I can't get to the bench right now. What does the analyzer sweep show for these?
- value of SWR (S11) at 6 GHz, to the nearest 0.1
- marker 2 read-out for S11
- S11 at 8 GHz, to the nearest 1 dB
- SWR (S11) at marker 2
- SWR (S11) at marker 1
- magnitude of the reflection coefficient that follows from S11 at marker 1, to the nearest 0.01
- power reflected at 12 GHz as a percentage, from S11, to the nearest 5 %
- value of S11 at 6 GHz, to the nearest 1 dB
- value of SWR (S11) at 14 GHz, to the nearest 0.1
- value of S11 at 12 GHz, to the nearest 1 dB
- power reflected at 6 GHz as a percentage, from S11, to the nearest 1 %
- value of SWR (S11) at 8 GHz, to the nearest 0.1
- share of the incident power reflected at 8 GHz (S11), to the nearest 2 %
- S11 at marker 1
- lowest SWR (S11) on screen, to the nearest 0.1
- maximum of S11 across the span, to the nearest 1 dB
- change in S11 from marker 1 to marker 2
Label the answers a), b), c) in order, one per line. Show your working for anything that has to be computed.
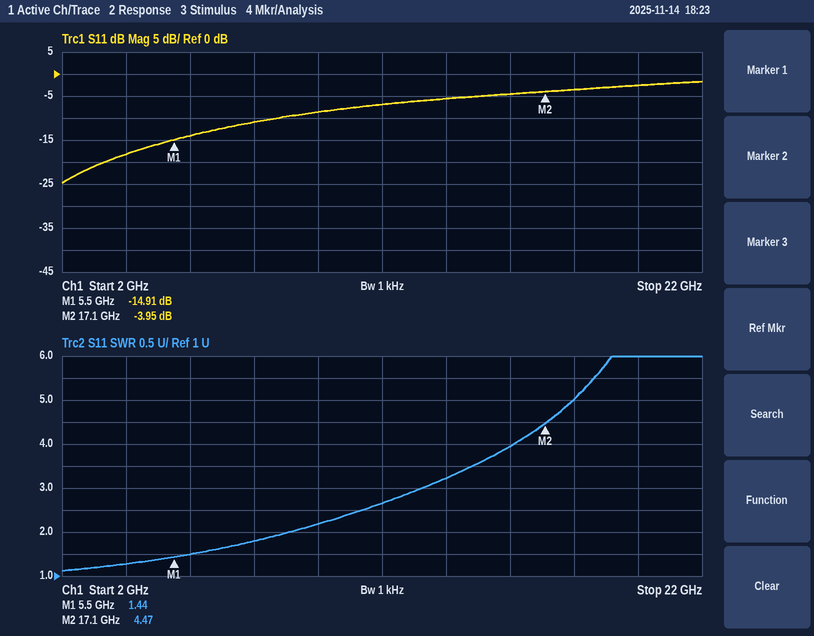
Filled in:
a) 1.5
b) -3.95 dB
c) -11 dB
d) 4.47
e) 1.44
f) 10^(-14.91/20) ≈ 0.18
g) 10^(-7/10) ≈ 20 %
h) -14 dB
i) 3.2
j) -7 dB
k) 10^(-14/10) ≈ 4 %
l) 1.8
m) 10^(-11/10) ≈ 8 %
n) -14.91 dB
o) 1.1
p) -2 dB
q) -3.95 − (-14.91) = 10.96 dB
